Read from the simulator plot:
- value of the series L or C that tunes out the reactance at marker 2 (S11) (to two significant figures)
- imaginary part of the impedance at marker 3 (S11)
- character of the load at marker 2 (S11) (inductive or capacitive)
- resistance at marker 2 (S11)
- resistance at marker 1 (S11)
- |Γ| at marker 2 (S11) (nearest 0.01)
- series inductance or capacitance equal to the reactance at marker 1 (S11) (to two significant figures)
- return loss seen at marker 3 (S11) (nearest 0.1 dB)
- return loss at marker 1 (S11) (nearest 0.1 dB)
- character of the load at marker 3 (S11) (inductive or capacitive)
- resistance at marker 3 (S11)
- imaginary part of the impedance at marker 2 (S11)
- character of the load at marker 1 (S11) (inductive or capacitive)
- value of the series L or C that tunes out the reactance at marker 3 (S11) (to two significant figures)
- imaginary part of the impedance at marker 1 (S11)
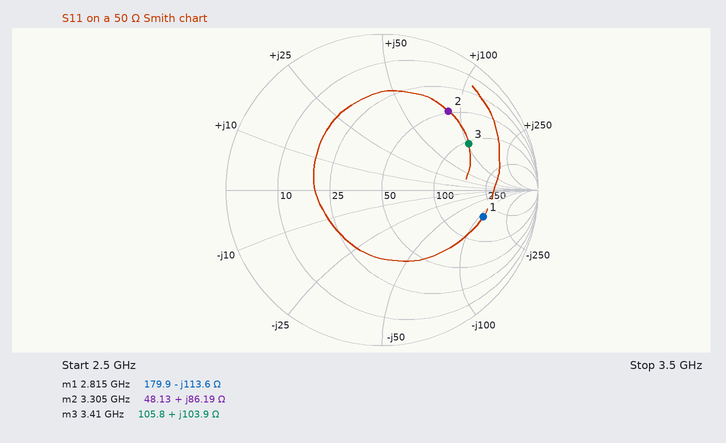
560 fF
+103.9 Ω
inductive
48.13 Ω
179.9 Ω
0.66
500 fF
4.0 dB
3.4 dB
inductive
105.8 Ω
+86.19 Ω
capacitive
450 fF
-113.6 Ω
